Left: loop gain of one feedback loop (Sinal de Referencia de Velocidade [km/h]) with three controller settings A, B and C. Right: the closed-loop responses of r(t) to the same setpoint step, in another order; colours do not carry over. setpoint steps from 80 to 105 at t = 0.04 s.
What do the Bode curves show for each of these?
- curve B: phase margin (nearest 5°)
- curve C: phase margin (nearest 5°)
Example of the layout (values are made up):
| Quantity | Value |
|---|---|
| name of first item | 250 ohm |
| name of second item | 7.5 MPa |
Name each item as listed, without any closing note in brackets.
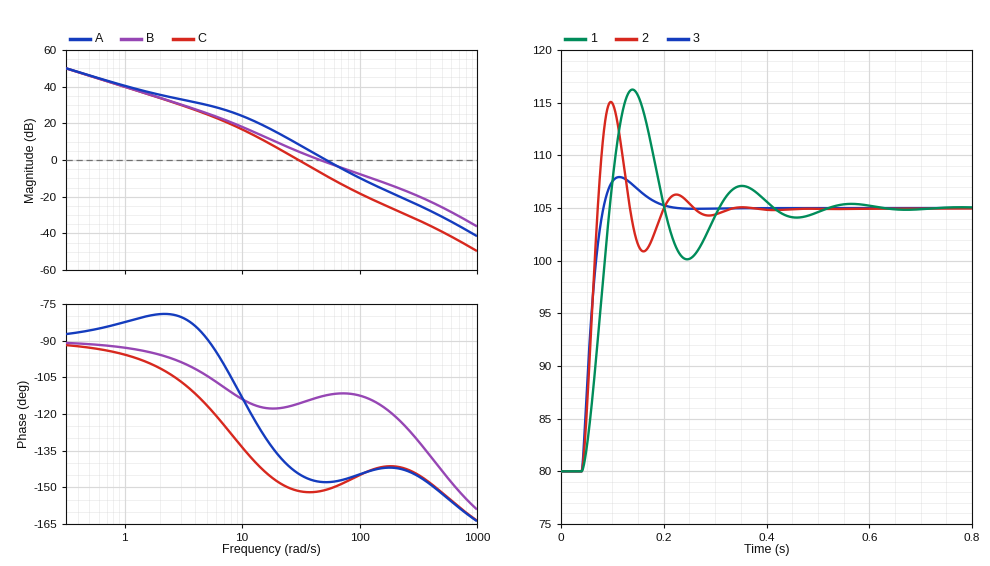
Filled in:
| Quantity | Value |
|---|---|
| curve B: phase margin | 65° |
| curve C: phase margin | 30° |
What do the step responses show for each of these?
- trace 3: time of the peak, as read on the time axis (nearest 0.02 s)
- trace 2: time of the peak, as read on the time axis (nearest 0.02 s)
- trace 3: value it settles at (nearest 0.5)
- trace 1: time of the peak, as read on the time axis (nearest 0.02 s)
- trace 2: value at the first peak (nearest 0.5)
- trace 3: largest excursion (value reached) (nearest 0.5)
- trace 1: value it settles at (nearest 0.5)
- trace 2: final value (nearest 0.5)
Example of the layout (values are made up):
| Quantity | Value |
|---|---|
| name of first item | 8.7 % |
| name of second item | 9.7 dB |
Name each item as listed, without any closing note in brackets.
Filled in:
| Quantity | Value |
|---|---|
| trace 3: time of the peak, as read on the time axis | 0.12 s |
| trace 2: time of the peak, as read on the time axis | 0.10 s |
| trace 3: value it settles at | 105.0 |
| trace 1: time of the peak, as read on the time axis | 0.14 s |
| trace 2: value at the first peak | 115.0 |
| trace 3: largest excursion (value reached) | 108.0 |
| trace 1: value it settles at | 105.0 |
| trace 2: final value | 105.0 |
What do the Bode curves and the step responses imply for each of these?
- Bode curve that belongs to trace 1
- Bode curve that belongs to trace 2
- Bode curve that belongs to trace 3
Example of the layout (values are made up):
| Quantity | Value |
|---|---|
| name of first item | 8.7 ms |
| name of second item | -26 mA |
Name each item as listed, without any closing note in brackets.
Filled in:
| Quantity | Value |
|---|---|
| Bode curve that belongs to trace 1 | C |
| Bode curve that belongs to trace 2 | A |
| Bode curve that belongs to trace 3 | B |
